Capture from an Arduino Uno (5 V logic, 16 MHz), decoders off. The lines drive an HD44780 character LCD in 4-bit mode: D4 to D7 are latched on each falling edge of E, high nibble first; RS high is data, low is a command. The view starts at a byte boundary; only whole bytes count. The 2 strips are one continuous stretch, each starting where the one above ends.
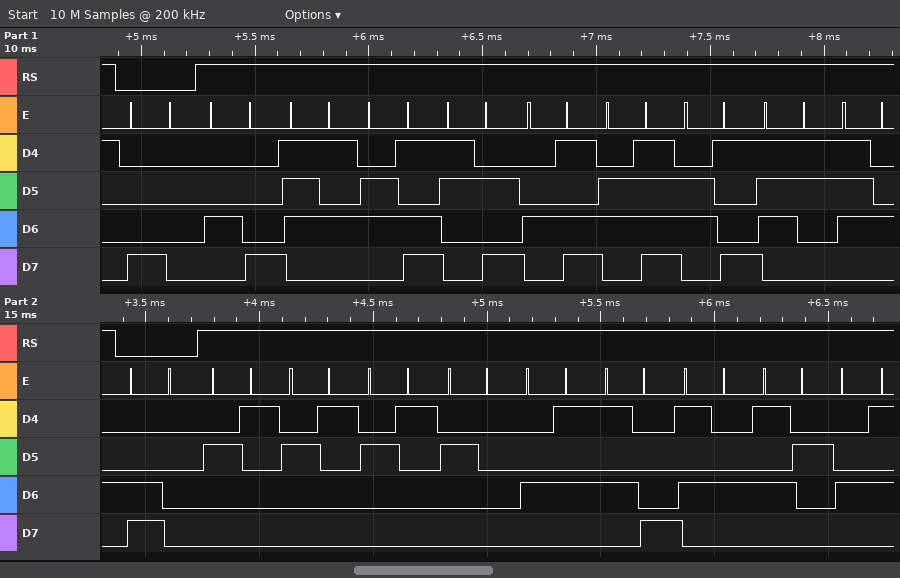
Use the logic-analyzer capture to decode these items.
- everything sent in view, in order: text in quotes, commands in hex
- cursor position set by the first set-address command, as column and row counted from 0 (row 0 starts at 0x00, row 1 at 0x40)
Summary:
0x80 "Hum:Moist" 0xC0 "!!! EXTRE"
column 0, row 0
